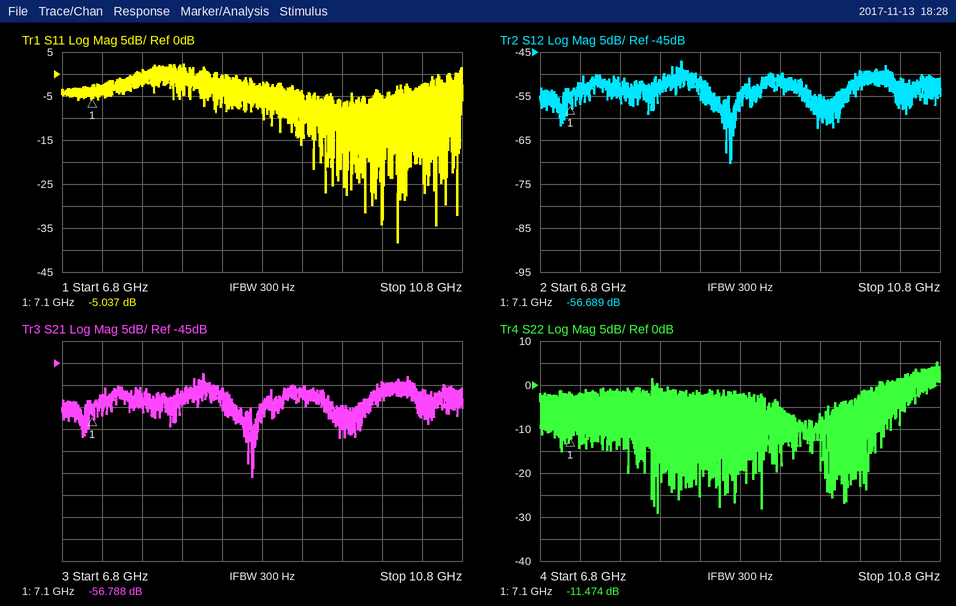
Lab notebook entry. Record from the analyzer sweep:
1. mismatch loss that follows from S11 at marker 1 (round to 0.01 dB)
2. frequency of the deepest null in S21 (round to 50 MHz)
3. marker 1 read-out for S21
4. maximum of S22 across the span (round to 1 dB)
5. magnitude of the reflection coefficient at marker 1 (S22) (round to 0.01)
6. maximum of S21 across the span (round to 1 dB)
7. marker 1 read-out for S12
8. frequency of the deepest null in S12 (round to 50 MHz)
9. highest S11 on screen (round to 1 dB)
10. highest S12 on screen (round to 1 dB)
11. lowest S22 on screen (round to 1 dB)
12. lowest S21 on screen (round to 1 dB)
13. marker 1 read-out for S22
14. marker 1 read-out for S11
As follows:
1.63 dB
8.70 GHz
-56.788 dB
5 dB
0.27
-47 dB
-56.689 dB
8.70 GHz
2 dB
-47 dB
-29 dB
-71 dB
-11.474 dB
-5.037 dB
